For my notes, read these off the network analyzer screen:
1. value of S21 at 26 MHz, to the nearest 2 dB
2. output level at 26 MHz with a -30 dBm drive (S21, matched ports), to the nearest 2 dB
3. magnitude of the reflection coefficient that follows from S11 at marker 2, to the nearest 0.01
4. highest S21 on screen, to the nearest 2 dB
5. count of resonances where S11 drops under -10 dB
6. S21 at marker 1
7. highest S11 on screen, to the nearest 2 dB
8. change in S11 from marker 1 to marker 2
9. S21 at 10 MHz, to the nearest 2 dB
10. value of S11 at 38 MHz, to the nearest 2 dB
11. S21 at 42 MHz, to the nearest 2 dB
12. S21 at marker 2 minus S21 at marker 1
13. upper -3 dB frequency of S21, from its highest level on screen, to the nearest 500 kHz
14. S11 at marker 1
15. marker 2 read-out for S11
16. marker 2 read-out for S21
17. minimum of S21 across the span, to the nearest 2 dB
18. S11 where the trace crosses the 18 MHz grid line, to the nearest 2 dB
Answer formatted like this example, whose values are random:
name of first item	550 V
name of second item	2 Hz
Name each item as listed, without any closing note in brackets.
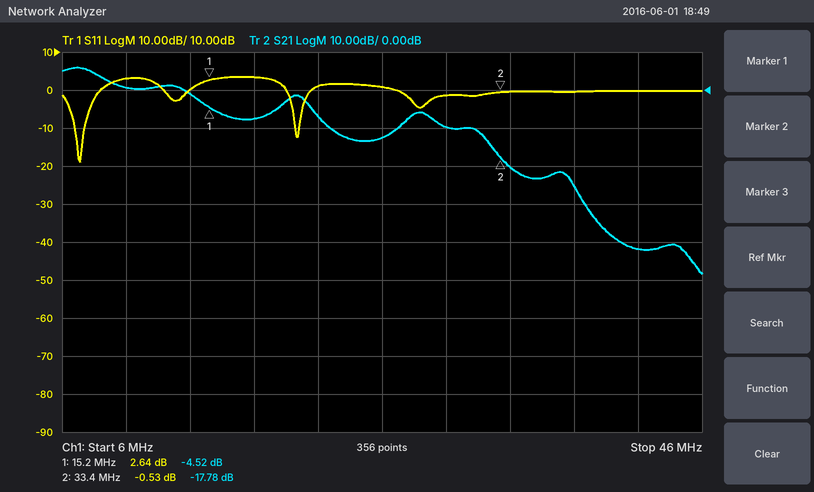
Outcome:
value of S21 at 26 MHz, to the nearest 2 dB	-12 dB
output level at 26 MHz with a -30 dBm drive (S21, matched ports), to the nearest 2 dB	-42 dBm
magnitude of the reflection coefficient that follows from S11 at marker 2, to the nearest 0.01	0.94
highest S21 on screen, to the nearest 2 dB	6 dB
count of resonances where S11 drops under -10 dB	2
S21 at marker 1	-4.52 dB
highest S11 on screen, to the nearest 2 dB	4 dB
change in S11 from marker 1 to marker 2	-3.17 dB
S21 at 10 MHz, to the nearest 2 dB	0 dB
value of S11 at 38 MHz, to the nearest 2 dB	0 dB
S21 at 42 MHz, to the nearest 2 dB	-42 dB
S21 at marker 2 minus S21 at marker 1	-13.26 dB
upper -3 dB frequency of S21, from its highest level on screen, to the nearest 500 kHz	8.5 MHz
S11 at marker 1	2.64 dB
marker 2 read-out for S11	-0.53 dB
marker 2 read-out for S21	-17.78 dB
minimum of S21 across the span, to the nearest 2 dB	-48 dB
S11 where the trace crosses the 18 MHz grid line, to the nearest 2 dB	4 dB
